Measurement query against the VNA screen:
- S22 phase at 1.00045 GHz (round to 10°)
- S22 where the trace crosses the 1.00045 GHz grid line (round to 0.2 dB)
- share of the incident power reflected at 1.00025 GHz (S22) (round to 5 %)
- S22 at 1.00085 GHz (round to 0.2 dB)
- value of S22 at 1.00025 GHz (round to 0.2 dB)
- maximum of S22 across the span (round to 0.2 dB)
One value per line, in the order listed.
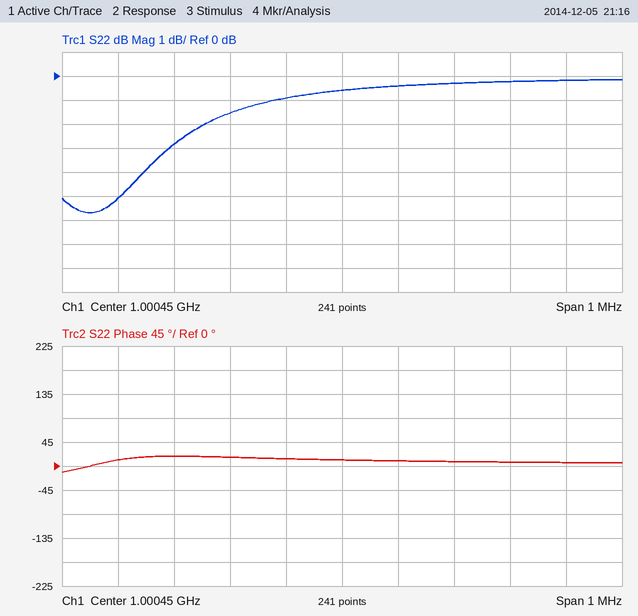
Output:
10°
-0.6 dB
70 %
-0.2 dB
-1.6 dB
-0.2 dB
